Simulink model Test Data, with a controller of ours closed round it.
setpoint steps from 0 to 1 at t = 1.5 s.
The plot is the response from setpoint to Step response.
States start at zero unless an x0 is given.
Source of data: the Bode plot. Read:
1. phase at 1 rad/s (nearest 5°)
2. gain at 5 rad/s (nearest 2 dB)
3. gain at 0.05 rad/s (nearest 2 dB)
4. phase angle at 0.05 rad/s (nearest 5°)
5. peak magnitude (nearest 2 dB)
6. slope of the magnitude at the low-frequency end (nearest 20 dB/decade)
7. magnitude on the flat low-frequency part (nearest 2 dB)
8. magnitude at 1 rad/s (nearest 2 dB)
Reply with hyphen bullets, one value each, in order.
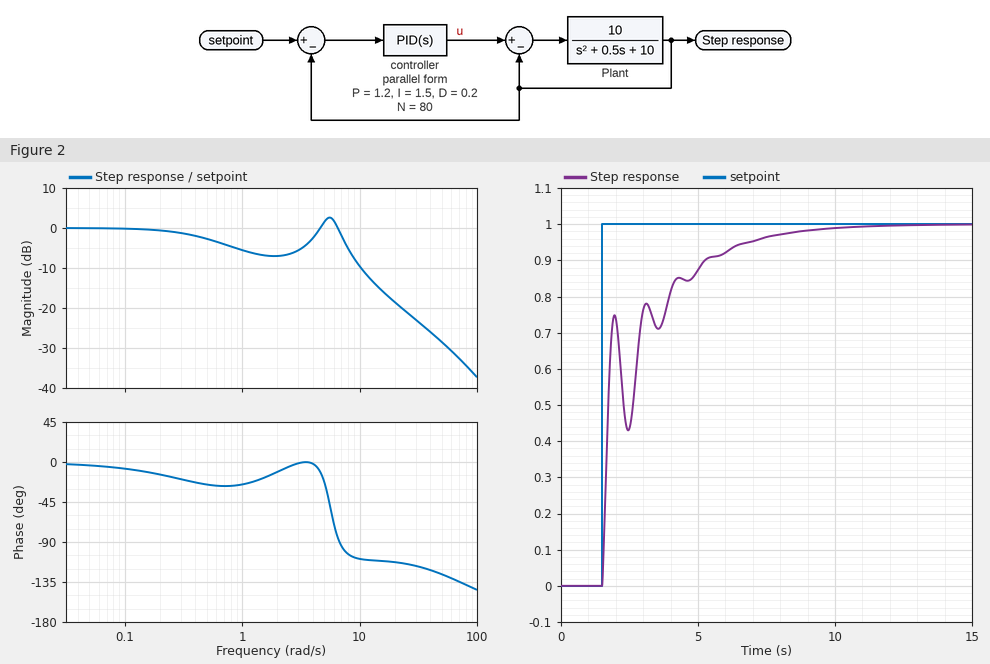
- -25°
- 2 dB
- 0 dB
- -5°
- 2 dB
- 0 dB/decade
- 0 dB
- -6 dB
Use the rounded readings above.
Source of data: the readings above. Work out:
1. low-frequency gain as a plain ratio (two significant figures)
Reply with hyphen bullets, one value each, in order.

- 1.0
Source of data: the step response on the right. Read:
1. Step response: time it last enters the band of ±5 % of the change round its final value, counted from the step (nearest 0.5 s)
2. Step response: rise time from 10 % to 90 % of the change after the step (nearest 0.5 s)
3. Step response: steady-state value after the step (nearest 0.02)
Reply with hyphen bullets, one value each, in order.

- 5.5 s
- 3.5 s
- 1.00
